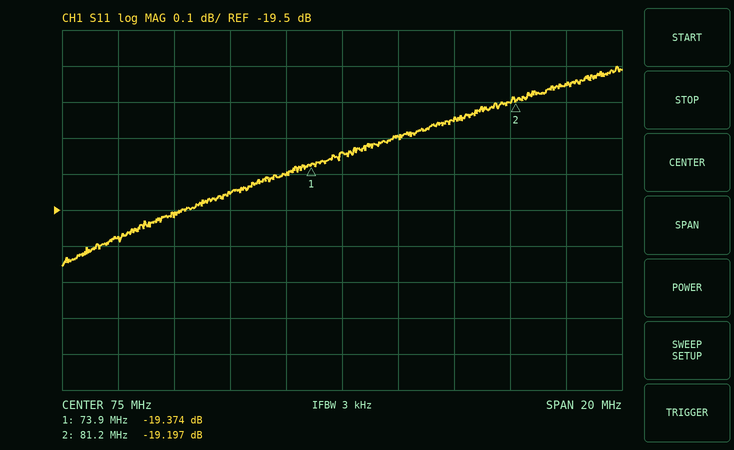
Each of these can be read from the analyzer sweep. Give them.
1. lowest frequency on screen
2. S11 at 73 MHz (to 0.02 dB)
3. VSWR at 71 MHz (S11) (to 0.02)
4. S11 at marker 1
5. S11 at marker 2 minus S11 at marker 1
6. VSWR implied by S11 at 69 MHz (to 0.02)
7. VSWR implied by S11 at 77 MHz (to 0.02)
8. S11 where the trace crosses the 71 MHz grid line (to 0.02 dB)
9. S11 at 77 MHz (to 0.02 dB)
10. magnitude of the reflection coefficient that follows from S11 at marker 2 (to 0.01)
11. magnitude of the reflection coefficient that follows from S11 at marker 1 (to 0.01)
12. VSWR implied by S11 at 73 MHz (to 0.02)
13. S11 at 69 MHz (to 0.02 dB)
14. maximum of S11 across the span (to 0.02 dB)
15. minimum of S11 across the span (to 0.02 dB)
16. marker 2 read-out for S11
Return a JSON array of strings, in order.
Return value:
["65 MHz", "-19.40 dB", "1.24", "-19.374 dB", "0.177 dB", "1.24", "1.24", "-19.46 dB", "-19.30 dB", "0.11", "0.11", "1.24", "-19.52 dB", "-19.10 dB", "-19.66 dB", "-19.197 dB"]
